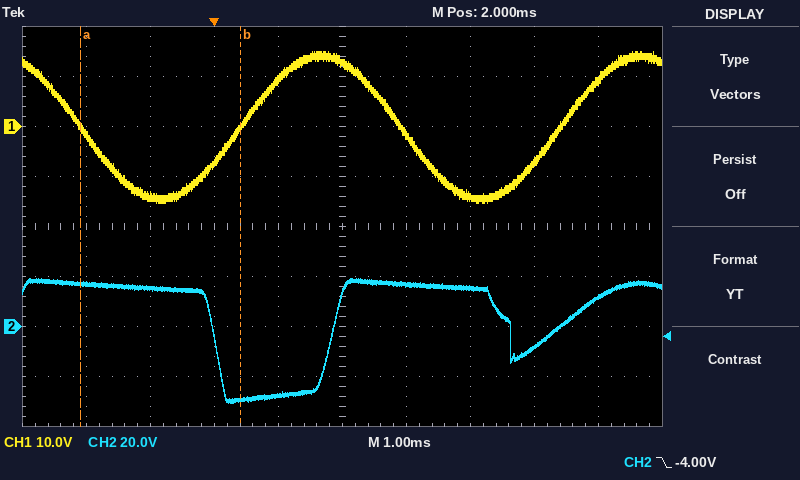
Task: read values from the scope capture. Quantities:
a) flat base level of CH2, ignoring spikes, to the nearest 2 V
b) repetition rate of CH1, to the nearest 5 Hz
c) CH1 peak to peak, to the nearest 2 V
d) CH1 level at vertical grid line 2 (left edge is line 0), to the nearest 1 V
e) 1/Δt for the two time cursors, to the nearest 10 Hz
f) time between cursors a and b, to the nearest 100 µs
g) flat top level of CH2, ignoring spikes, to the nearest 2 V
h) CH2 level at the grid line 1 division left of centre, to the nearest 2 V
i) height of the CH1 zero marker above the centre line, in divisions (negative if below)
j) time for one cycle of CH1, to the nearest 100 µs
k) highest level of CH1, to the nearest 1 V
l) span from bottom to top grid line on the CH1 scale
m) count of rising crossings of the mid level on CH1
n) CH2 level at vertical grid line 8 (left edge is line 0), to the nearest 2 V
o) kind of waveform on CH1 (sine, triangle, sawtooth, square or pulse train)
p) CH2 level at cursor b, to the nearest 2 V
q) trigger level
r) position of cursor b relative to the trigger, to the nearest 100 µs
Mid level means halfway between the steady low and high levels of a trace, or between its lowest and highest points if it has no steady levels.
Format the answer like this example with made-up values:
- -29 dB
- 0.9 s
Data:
- -28 V
- 200 Hz
- 30 V
- -14 V
- 400 Hz
- 2.5 ms
- 16 V
- -28 V
- +2.0 div
- 5.0 ms
- 15 V
- 80 V
- 2
- -8 V
- sine
- -30 V
- -4.00 V
- +400 µs
